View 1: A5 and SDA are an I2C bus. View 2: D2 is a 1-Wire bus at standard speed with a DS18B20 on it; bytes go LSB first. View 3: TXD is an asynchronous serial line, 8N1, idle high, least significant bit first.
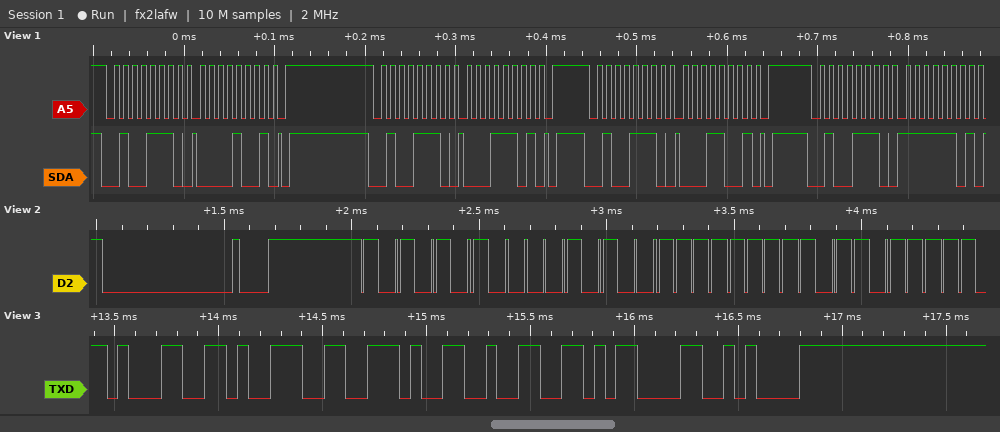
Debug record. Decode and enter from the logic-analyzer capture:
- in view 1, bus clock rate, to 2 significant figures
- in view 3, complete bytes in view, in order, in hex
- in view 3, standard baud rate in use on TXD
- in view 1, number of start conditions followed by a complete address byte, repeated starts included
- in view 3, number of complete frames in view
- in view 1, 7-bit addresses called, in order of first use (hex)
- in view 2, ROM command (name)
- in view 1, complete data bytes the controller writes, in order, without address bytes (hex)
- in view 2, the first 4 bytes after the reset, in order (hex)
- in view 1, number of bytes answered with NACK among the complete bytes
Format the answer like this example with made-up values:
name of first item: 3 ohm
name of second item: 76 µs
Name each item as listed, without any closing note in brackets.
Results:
in view 1, bus clock rate, to 2 significant figures: 100 kHz
in view 3, complete bytes in view, in order, in hex: 31 39 2E 32 0D 0A
in view 3, standard baud rate in use on TXD: 19200 baud
in view 1, number of start conditions followed by a complete address byte, repeated starts included: 4
in view 3, number of complete frames in view: 6
in view 1, 7-bit addresses called, in order of first use: 0x27
in view 2, ROM command: Match ROM
in view 1, complete data bytes the controller writes, in order, without address bytes: 09 1D 19 FD
in view 2, the first 4 bytes after the reset, in order: 55 28 FF ED
in view 1, number of bytes answered with NACK among the complete bytes: 0
